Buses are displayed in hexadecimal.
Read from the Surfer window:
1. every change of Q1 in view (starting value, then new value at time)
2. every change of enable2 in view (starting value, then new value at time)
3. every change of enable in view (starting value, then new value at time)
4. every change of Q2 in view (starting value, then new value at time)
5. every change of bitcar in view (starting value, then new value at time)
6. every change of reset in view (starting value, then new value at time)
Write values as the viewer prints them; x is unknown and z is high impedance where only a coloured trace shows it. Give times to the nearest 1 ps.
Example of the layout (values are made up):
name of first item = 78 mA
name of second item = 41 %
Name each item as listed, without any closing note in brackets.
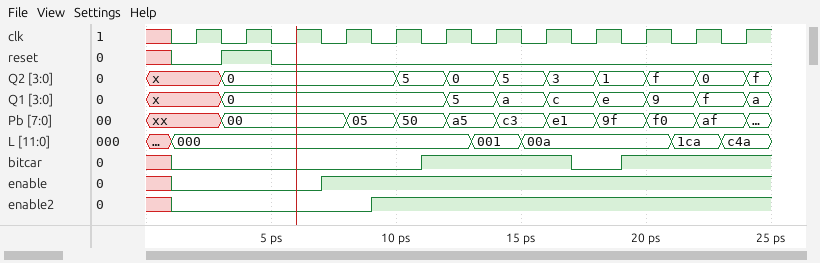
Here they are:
every change of Q1 in view = x, 0 at 3 ps, 5 at 12 ps, a at 14 ps, c at 16 ps, e at 18 ps, 9 at 20 ps, f at 22 ps, a at 24 ps
every change of enable2 in view = x, 0 at 1 ps, 1 at 9 ps
every change of enable in view = x, 0 at 1 ps, 1 at 7 ps
every change of Q2 in view = x, 0 at 3 ps, 5 at 10 ps, 0 at 12 ps, 5 at 14 ps, 3 at 16 ps, 1 at 18 ps, f at 20 ps, 0 at 22 ps, f at 24 ps
every change of bitcar in view = x, 0 at 1 ps, 1 at 11 ps, 0 at 17 ps, 1 at 19 ps
every change of reset in view = x, 0 at 1 ps, 1 at 3 ps, 0 at 5 ps
